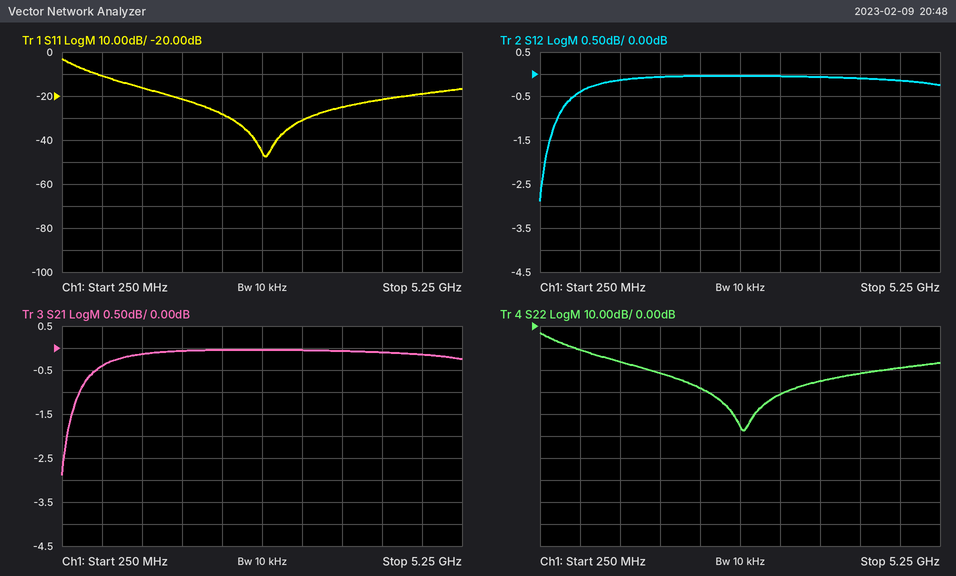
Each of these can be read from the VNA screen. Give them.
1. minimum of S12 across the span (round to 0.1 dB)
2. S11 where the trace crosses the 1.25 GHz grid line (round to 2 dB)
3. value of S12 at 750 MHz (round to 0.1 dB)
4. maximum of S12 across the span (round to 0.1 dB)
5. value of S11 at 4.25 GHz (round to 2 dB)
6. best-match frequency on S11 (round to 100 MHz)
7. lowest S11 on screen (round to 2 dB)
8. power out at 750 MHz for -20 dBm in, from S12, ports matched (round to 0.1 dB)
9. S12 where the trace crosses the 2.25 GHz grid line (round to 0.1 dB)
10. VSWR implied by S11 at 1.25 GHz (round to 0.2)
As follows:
-2.9 dB
-16 dB
-0.4 dB
0.0 dB
-22 dB
2.8 GHz
-48 dB
-20.4 dBm
0.0 dB
1.4
